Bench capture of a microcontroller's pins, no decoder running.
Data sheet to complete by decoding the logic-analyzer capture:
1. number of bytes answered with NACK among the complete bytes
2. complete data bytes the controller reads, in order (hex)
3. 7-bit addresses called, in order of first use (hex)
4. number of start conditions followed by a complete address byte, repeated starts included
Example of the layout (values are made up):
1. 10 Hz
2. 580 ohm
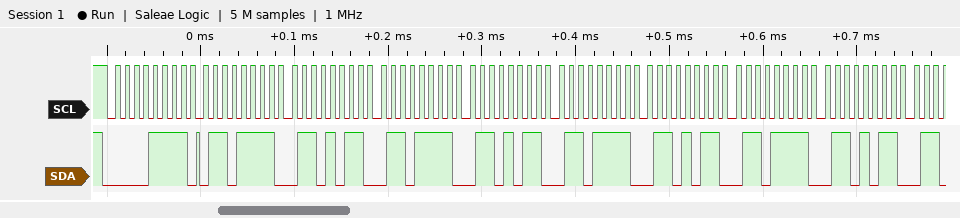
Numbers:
1. 0
2. 6F 6B 6F 6B 6F 6B 6F 6B
3. 0x07
4. 1
